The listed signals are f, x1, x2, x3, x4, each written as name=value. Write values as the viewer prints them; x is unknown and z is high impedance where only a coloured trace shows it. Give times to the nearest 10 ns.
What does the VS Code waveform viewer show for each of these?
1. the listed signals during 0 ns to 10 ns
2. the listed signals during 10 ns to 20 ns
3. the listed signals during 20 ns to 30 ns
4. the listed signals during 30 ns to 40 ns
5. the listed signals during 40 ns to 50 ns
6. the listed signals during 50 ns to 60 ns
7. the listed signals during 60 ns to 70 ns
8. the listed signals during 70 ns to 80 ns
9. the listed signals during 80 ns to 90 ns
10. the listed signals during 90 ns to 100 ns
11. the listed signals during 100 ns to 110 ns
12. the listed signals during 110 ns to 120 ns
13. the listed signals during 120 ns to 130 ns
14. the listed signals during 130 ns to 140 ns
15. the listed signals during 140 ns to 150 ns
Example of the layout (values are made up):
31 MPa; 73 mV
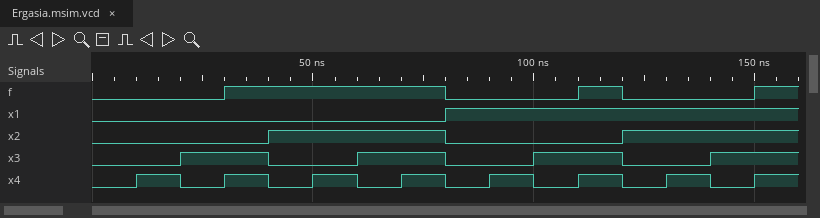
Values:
f=0, x1=0, x2=0, x3=0, x4=0; f=0, x1=0, x2=0, x3=0, x4=1; f=0, x1=0, x2=0, x3=1, x4=0; f=1, x1=0, x2=0, x3=1, x4=1; f=1, x1=0, x2=1, x3=0, x4=0; f=1, x1=0, x2=1, x3=0, x4=1; f=1, x1=0, x2=1, x3=1, x4=0; f=1, x1=0, x2=1, x3=1, x4=1; f=0, x1=1, x2=0, x3=0, x4=0; f=0, x1=1, x2=0, x3=0, x4=1; f=0, x1=1, x2=0, x3=1, x4=0; f=1, x1=1, x2=0, x3=1, x4=1; f=0, x1=1, x2=1, x3=0, x4=0; f=0, x1=1, x2=1, x3=0, x4=1; f=0, x1=1, x2=1, x3=1, x4=0
